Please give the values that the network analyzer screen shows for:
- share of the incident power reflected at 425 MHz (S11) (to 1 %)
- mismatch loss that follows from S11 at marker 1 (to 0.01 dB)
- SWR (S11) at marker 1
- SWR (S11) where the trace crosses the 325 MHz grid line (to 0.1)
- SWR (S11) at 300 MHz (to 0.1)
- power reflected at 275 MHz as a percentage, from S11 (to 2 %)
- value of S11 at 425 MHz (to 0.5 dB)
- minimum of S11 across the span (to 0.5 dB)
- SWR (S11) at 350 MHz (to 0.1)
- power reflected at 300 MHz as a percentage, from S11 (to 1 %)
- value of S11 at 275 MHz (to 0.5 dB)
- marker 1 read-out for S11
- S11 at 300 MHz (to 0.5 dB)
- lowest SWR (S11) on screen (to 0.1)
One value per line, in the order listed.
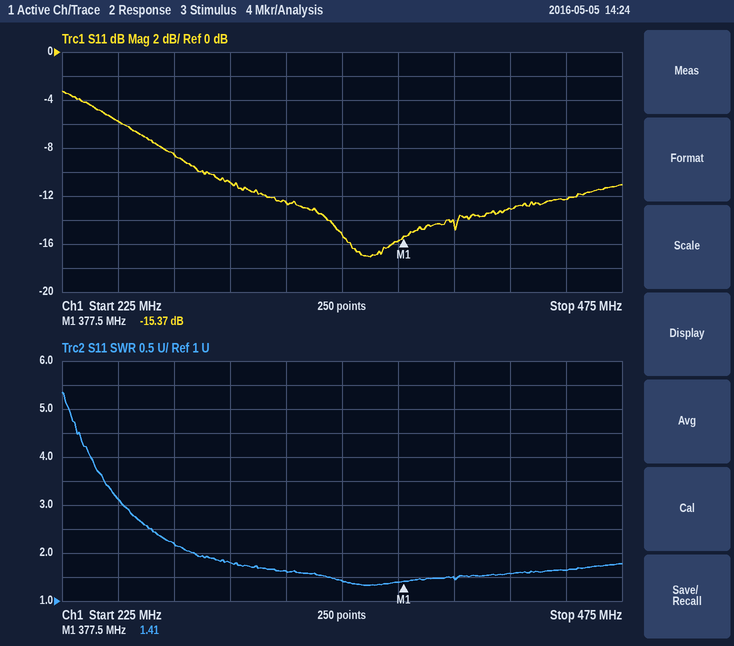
5 %
0.13 dB
1.41
1.6
1.8
14 %
-13.0 dB
-17.0 dB
1.4
8 %
-8.5 dB
-15.37 dB
-11.0 dB
1.3
